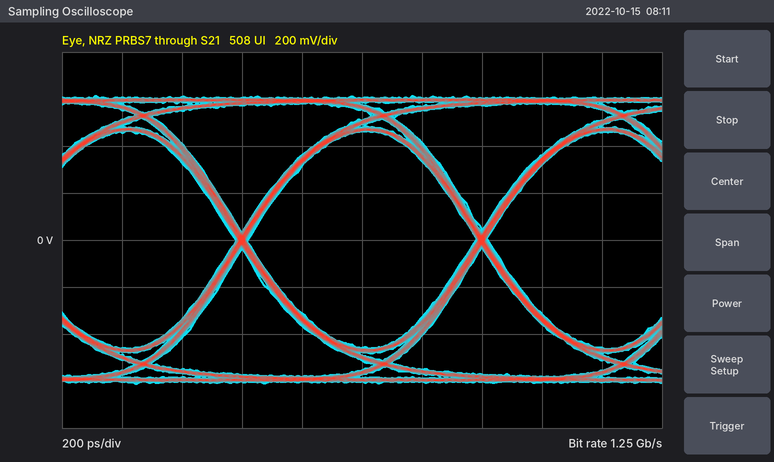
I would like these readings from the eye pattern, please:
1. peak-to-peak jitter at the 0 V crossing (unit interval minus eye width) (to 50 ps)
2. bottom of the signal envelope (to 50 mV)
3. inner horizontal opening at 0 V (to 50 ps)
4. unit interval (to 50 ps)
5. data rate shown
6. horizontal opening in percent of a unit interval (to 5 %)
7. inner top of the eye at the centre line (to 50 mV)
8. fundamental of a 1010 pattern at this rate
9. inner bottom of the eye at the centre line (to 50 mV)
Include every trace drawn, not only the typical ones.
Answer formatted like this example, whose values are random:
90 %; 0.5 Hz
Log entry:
50 ps; -600 mV; 750 ps; 800 ps; 1.25 Gb/s; 95 %; 450 mV; 625 MHz; -450 mV
